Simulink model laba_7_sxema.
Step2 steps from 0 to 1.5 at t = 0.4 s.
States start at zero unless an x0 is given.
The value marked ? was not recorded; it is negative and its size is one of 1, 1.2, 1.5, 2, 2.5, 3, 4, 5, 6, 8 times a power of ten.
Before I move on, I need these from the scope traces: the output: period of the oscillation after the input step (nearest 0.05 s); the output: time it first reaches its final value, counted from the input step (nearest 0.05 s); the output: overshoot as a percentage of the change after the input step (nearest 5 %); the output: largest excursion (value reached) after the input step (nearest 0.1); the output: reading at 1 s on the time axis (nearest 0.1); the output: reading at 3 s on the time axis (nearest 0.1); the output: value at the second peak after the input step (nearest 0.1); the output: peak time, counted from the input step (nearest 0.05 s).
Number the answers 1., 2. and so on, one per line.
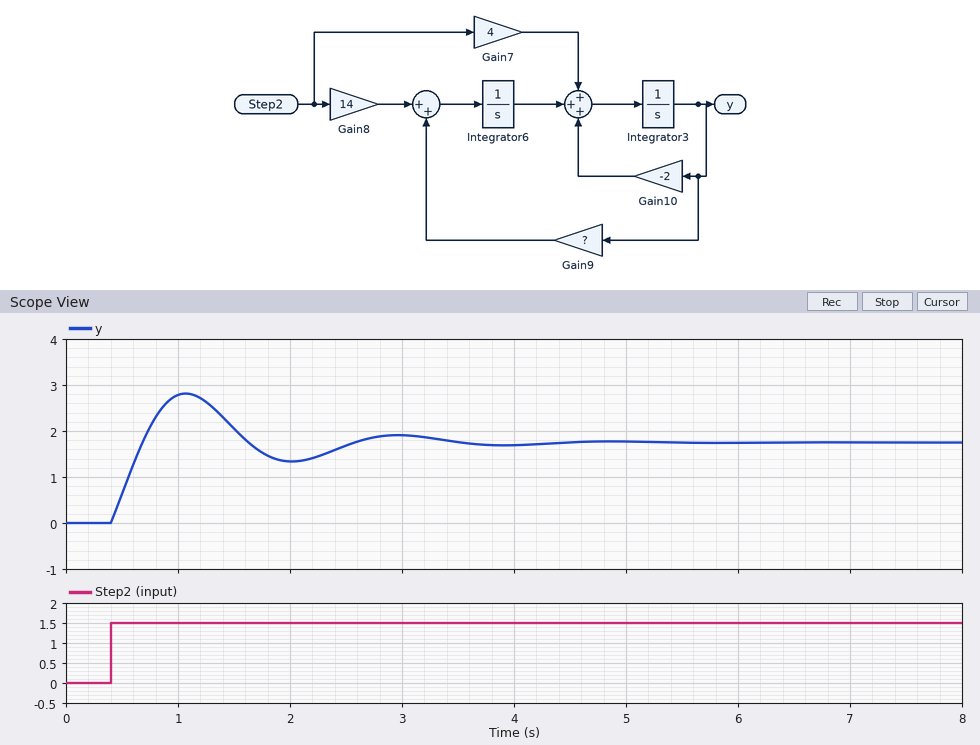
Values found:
1. 1.90 s
2. 0.30 s
3. 60 %
4. 2.8
5. 2.8
6. 1.9
7. 1.9
8. 0.65 s
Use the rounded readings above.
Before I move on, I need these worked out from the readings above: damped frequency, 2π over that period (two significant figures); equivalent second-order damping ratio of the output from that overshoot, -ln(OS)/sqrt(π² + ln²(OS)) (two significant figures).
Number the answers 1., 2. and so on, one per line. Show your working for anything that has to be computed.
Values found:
1. 2π / 1.9 = 3.3 rad/s
2. ln(0.6) = -0.511; 0.511 / sqrt(9.870 + 0.261) = 0.16
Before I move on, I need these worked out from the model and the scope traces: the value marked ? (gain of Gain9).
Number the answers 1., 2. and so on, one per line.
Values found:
1. -12
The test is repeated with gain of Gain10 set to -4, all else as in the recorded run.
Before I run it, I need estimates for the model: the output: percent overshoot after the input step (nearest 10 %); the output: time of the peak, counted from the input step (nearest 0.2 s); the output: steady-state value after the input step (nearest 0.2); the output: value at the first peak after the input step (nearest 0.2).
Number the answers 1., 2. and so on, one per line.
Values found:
1. 20 %
2. 0.8 s
3. 1.8
4. 2.2
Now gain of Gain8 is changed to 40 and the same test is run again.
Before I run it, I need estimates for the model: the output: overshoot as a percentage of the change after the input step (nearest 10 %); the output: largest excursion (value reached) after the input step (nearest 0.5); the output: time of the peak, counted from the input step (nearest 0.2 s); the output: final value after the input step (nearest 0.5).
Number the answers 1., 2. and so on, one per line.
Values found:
1. 40 %
2. 7.0
3. 0.8 s
4. 5.0
